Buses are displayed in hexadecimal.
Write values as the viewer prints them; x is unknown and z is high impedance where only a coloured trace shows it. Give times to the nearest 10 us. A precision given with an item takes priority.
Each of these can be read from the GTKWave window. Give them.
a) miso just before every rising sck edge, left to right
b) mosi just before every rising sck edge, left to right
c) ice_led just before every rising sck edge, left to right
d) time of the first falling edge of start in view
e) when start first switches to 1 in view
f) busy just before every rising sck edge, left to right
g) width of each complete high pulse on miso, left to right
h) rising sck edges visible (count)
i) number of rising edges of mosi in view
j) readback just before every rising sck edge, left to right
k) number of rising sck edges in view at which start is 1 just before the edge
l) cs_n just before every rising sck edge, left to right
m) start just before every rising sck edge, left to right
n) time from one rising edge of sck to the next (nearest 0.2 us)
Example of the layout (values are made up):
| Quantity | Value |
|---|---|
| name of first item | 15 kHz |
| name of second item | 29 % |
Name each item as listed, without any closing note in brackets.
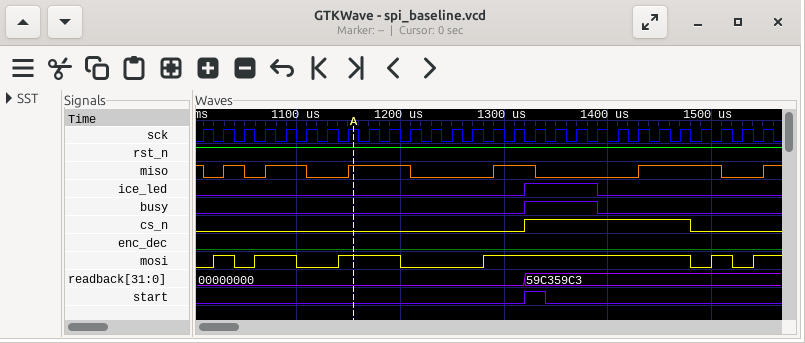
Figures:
| Quantity | Value |
|---|---|
| miso just before every rising sck edge, left to right | 1 0 1 0 1 1 0 0 1 1 1 0 0 0 0 1 1 0 0 0 0 0 1 1 1 1 0 0 |
| mosi just before every rising sck edge, left to right | 0 1 0 1 1 0 0 1 1 1 0 0 0 0 1 1 1 1 1 1 1 1 1 1 0 1 0 1 |
| ice_led just before every rising sck edge, left to right | 0 0 0 0 0 0 0 0 0 0 0 0 0 0 0 0 1 1 1 1 0 0 0 0 0 0 0 0 |
| time of the first falling edge of start in view | 1340 us |
| when start first switches to 1 in view | 1320 us |
| busy just before every rising sck edge, left to right | 0 0 0 0 0 0 0 0 0 0 0 0 0 0 0 0 1 1 1 1 0 0 0 0 0 0 0 0 |
| width of each complete high pulse on miso, left to right | 20 us, 40 us, 60 us, 40 us, 80 us |
| rising sck edges visible | 28 |
| number of rising edges of mosi in view | 6 |
| readback just before every rising sck edge, left to right | 00000000, 00000000, 00000000, 00000000, 00000000, 00000000, 00000000, 00000000, 00000000, 00000000, 00000000, 00000000, 00000000, 00000000, 00000000, 00000000, 59C359C3, 59C359C3, 59C359C3, 59C359C3, 59C359C3, 59C359C3, 59C359C3, 59C359C3, 59C359C3, 59C359C3, 59C359C3, 59C359C3 |
| number of rising sck edges in view at which start is 1 just before the edge | 1 |
| cs_n just before every rising sck edge, left to right | 0 0 0 0 0 0 0 0 0 0 0 0 0 0 0 0 1 1 1 1 1 1 1 1 0 0 0 0 |
| start just before every rising sck edge, left to right | 0 0 0 0 0 0 0 0 0 0 0 0 0 0 0 0 1 0 0 0 0 0 0 0 0 0 0 0 |
| time from one rising edge of sck to the next | 20 us |
